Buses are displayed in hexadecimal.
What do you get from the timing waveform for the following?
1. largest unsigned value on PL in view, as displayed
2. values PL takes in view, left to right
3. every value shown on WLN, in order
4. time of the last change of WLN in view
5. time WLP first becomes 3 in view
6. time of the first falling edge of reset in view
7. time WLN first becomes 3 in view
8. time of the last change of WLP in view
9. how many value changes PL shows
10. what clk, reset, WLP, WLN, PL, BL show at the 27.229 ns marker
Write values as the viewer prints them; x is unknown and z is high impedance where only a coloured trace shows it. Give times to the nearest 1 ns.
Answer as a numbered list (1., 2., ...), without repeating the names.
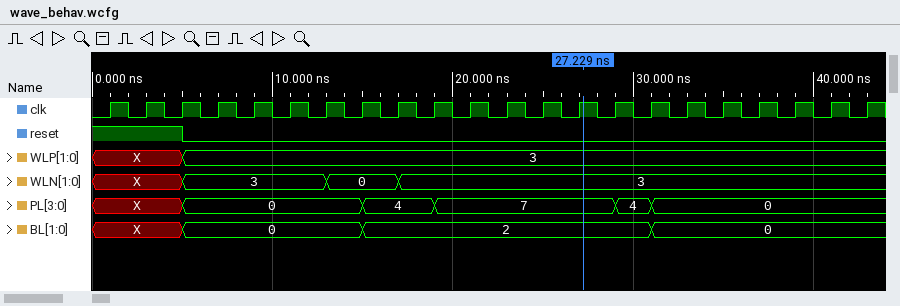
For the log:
1. 7
2. X, 0, 4, 7, 4, 0
3. X, 3, 0, 3
4. 17 ns
5. 5 ns
6. 5 ns
7. 5 ns
8. 5 ns
9. 5
10. clk=1, reset=0, WLP=3, WLN=3, PL=7, BL=2
